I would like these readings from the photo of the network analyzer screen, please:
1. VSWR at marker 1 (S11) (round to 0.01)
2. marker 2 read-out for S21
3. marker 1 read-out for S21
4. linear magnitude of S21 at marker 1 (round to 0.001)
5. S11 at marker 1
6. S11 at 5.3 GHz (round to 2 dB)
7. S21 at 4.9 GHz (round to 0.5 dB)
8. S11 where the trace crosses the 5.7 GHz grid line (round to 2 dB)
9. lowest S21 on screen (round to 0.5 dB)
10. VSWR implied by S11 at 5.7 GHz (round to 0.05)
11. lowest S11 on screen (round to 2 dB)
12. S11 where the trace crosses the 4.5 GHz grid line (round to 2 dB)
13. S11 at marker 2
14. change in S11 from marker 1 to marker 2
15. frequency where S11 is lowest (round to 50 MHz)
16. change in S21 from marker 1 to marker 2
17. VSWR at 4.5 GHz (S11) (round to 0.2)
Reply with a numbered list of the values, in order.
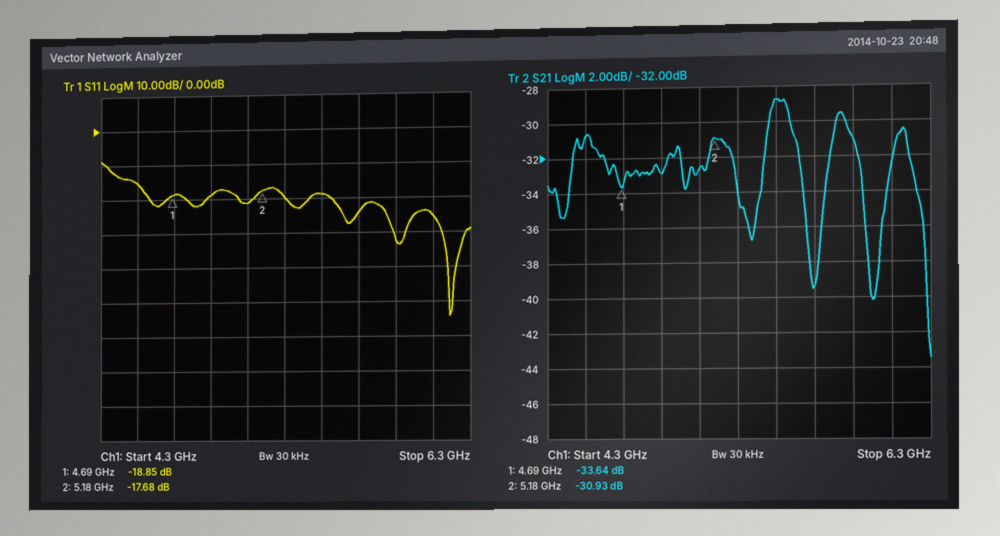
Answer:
1. 1.26
2. -30.93 dB
3. -33.64 dB
4. 0.021
5. -18.85 dB
6. -20 dB
7. -33.0 dB
8. -24 dB
9. -43.5 dB
10. 1.15
11. -54 dB
12. -16 dB
13. -17.68 dB
14. 1.17 dB
15. 6.20 GHz
16. 2.71 dB
17. 1.4
